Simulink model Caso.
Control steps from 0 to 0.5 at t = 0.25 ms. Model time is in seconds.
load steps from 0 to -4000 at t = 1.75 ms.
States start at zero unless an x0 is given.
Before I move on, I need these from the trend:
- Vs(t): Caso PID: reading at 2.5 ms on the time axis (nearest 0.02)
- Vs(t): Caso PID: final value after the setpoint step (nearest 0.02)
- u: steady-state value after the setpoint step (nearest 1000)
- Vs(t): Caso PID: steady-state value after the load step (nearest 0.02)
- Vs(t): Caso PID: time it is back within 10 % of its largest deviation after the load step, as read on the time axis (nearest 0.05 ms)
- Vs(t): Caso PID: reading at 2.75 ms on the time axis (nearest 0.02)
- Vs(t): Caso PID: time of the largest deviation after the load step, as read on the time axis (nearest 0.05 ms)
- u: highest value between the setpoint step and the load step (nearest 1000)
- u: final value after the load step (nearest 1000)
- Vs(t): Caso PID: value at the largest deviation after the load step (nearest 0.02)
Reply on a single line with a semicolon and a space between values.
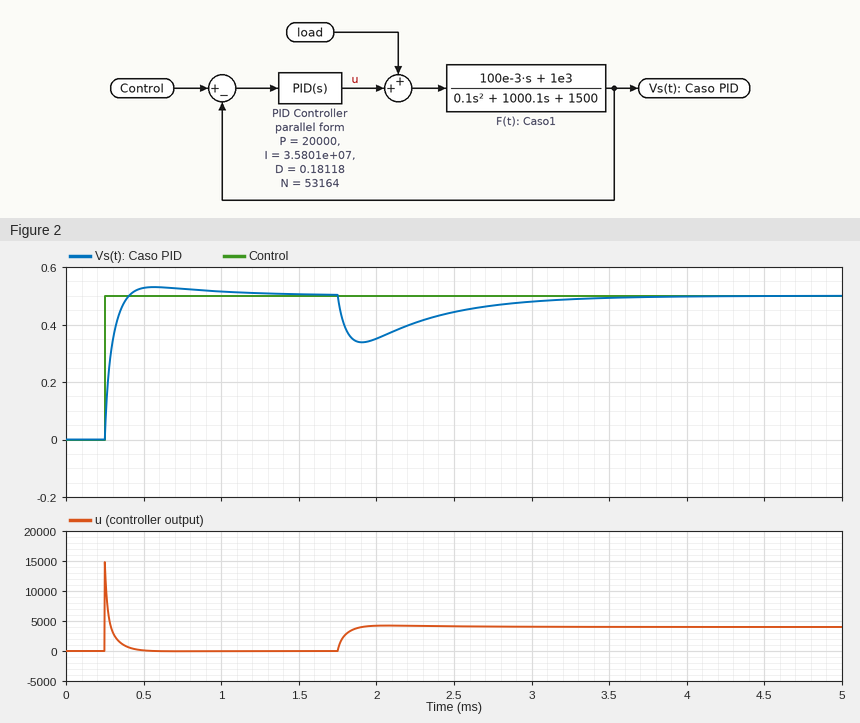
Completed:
0.44; 0.50; 0; 0.50; 3.10 ms; 0.46; 1.90 ms; 15000; 4000; 0.34
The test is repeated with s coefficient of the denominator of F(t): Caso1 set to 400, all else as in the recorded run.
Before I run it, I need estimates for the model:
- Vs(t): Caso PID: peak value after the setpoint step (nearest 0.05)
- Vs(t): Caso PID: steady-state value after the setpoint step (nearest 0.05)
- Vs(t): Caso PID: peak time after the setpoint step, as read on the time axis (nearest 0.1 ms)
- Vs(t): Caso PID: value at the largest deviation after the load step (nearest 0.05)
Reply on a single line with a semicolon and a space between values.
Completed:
0.55; 0.50; 0.4 ms; 0.30
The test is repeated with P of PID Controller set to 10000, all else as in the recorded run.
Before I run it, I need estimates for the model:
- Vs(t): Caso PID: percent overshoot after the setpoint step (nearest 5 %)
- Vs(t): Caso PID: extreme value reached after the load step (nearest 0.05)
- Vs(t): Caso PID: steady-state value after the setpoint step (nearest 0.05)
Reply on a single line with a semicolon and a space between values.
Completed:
15 %; 0.25; 0.50
